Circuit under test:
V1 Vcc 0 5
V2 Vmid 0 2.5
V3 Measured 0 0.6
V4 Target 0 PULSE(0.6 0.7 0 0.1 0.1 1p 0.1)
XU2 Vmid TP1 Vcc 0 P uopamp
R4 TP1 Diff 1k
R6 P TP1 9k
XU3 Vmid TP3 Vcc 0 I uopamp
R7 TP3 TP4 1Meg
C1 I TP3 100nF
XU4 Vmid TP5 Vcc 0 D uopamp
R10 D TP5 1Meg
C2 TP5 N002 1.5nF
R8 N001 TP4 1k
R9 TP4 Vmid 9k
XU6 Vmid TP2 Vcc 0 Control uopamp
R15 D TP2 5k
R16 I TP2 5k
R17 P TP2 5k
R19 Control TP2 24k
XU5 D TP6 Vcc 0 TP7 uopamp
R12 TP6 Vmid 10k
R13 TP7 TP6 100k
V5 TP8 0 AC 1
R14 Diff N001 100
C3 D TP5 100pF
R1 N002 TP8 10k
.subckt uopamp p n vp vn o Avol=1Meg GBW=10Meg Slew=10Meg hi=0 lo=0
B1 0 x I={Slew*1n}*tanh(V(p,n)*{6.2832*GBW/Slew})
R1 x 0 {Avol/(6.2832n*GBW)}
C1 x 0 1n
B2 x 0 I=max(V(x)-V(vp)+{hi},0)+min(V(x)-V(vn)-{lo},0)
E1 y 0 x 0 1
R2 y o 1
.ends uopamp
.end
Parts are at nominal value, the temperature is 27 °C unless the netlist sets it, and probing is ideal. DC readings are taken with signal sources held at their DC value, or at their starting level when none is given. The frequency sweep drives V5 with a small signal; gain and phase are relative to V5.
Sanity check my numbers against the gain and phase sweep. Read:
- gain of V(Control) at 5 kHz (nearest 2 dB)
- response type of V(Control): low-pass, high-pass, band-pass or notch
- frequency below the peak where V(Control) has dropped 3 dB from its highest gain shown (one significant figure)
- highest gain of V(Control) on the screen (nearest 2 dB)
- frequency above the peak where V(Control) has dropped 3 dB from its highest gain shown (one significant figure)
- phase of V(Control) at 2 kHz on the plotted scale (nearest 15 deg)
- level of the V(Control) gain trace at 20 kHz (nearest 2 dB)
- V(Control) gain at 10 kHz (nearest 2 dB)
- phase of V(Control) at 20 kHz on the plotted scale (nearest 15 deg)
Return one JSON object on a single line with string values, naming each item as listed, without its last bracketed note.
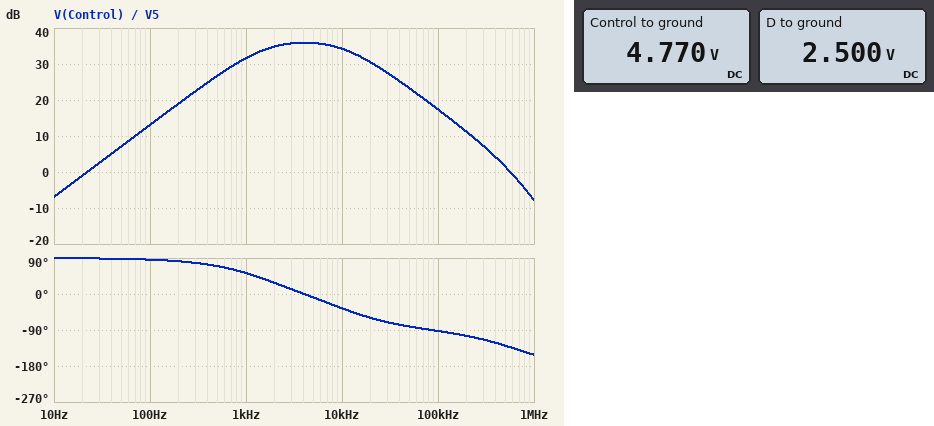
{"gain of V(Control) at 5 kHz": "36 dB", "response type of V(Control): low-pass, high-pass, band-pass or notch": "band-pass", "frequency below the peak where V(Control) has dropped 3 dB from its highest gain shown": "1 kHz", "highest gain of V(Control) on the screen": "36 dB", "frequency above the peak where V(Control) has dropped 3 dB from its highest gain shown": "10 kHz", "phase of V(Control) at 2 kHz on the plotted scale": "30 deg", "level of the V(Control) gain trace at 20 kHz": "30 dB", "V(Control) gain at 10 kHz": "34 dB", "phase of V(Control) at 20 kHz on the plotted scale": "-60 deg"}
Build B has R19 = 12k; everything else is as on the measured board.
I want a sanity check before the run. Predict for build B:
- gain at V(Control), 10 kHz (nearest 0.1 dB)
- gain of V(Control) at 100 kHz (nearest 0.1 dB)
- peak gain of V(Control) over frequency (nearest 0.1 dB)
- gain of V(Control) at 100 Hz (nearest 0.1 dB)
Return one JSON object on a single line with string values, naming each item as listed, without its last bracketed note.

{"gain at V(Control), 10 kHz": "28.2 dB", "gain of V(Control) at 100 kHz": "11.4 dB", "peak gain of V(Control) over frequency": "29.9 dB", "gain of V(Control) at 100 Hz": "7.1 dB"}
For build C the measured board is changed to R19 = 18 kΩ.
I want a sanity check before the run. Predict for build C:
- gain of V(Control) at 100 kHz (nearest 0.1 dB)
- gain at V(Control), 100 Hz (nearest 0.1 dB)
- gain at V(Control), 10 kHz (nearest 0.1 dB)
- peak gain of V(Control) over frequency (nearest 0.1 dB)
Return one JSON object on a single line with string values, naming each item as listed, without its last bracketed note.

{"gain of V(Control) at 100 kHz": "14.9 dB", "gain at V(Control), 100 Hz": "10.6 dB", "gain at V(Control), 10 kHz": "31.7 dB", "peak gain of V(Control) over frequency": "33.4 dB"}
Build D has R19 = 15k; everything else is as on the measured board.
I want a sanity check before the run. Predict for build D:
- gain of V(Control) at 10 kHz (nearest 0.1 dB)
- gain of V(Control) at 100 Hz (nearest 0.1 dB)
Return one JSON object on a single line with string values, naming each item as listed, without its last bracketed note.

{"gain of V(Control) at 10 kHz": "30.1 dB", "gain of V(Control) at 100 Hz": "9.0 dB"}
